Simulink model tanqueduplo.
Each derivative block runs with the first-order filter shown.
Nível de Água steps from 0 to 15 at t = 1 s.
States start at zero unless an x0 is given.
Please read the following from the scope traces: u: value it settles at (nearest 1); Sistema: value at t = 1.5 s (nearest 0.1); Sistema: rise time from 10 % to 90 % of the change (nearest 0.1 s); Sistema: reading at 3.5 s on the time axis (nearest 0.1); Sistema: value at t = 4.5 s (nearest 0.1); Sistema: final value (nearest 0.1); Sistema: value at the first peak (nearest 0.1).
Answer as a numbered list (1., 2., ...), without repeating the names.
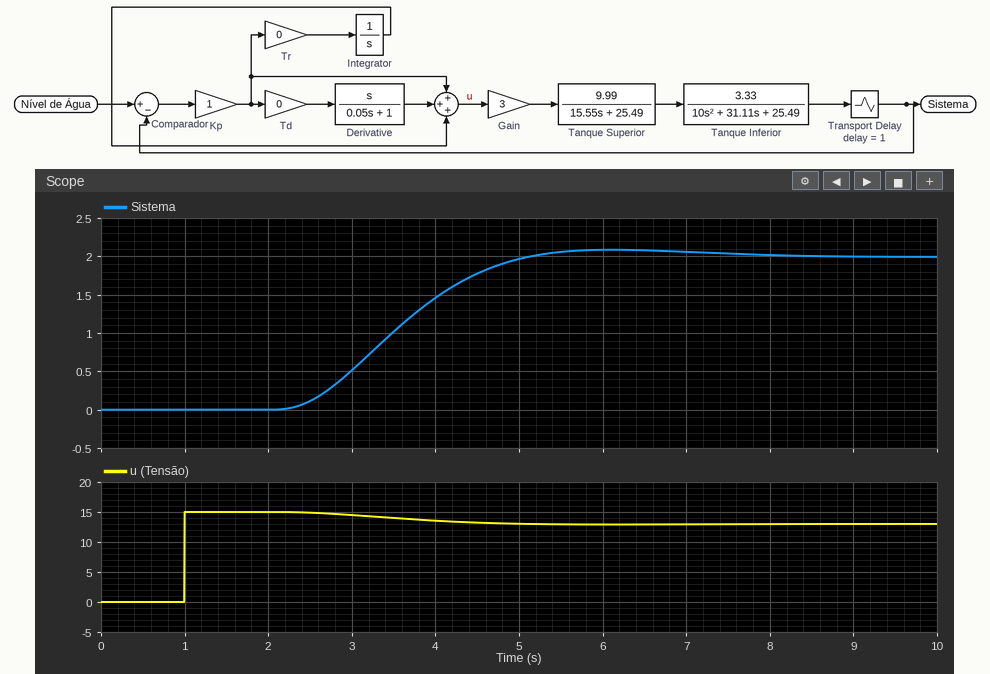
1. 13
2. 0.0
3. 1.9 s
4. 1.0
5. 1.8
6. 2.0
7. 2.1
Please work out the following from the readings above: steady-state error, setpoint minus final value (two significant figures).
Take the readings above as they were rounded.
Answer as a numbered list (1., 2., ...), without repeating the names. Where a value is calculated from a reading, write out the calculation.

1. 15 - 2 = 13
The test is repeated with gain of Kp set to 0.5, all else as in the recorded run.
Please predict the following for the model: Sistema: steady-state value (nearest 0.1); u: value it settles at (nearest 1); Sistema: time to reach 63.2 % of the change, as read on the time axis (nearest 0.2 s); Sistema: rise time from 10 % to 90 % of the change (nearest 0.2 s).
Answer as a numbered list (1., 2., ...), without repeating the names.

1. 1.1
2. 7
3. 3.8 s
4. 2.2 s
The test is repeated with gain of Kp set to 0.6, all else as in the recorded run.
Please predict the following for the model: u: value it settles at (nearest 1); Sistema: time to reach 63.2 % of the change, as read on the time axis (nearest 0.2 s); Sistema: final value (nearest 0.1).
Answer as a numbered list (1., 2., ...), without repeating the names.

1. 8
2. 3.8 s
3. 1.3
